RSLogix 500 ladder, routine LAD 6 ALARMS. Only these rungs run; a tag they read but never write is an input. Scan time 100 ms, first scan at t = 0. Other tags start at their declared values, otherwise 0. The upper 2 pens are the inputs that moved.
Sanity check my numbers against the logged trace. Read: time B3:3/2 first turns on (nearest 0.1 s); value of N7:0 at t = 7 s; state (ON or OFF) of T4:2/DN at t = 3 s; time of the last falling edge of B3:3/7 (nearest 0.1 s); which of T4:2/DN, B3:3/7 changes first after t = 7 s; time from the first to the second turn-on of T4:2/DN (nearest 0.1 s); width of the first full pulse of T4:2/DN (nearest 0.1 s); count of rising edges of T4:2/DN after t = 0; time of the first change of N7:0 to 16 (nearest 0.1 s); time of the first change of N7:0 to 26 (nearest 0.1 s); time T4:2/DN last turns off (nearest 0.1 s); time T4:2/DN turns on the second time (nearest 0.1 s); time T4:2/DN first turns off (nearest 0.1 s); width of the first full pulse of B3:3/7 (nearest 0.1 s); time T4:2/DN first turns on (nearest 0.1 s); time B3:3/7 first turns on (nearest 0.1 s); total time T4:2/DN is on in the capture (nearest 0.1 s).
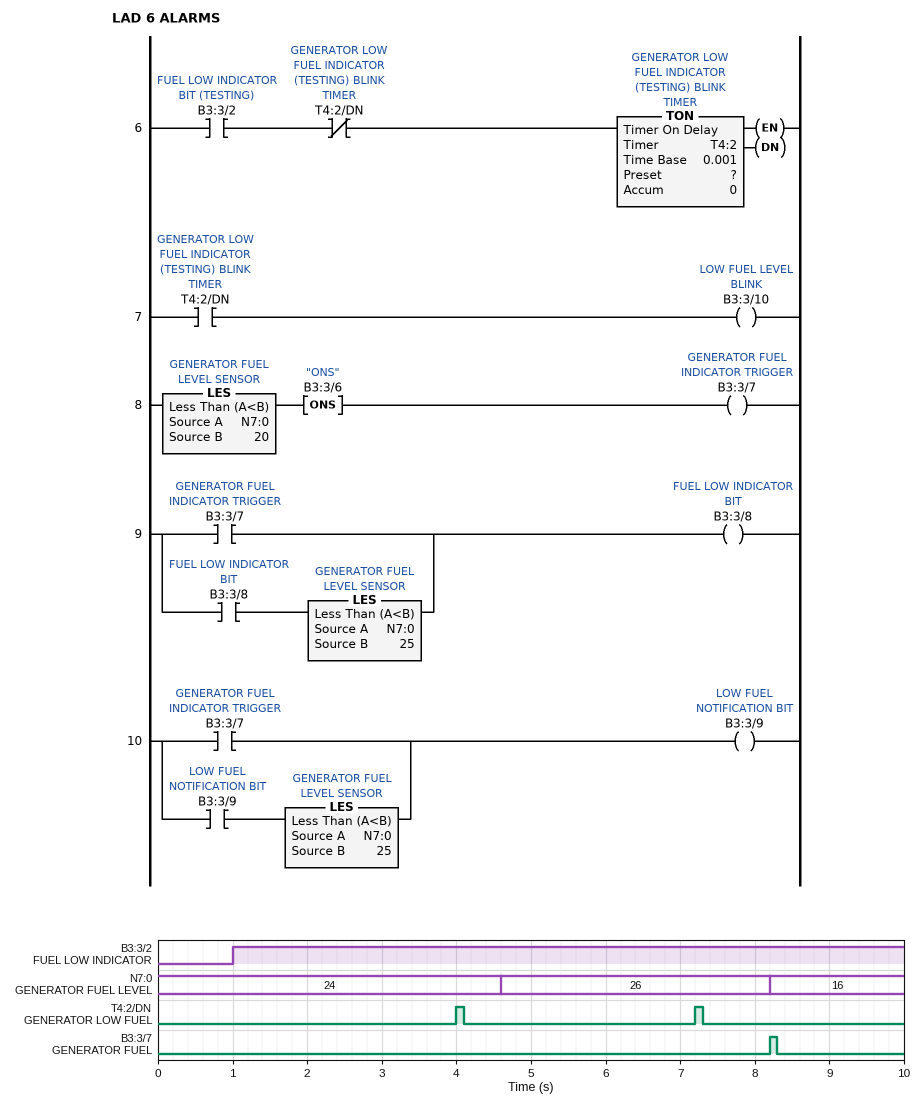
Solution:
1.0 s
26
OFF
8.3 s
T4:2/DN
3.2 s
0.1 s
2
8.2 s
4.6 s
7.3 s
7.2 s
4.1 s
0.1 s
4.0 s
8.2 s
0.2 s
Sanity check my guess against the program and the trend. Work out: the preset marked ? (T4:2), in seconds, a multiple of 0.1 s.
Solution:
3.0 s
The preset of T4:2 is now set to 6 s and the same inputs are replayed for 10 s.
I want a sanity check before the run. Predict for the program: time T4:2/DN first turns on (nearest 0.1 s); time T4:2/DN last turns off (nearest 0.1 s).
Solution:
7.0 s
7.1 s
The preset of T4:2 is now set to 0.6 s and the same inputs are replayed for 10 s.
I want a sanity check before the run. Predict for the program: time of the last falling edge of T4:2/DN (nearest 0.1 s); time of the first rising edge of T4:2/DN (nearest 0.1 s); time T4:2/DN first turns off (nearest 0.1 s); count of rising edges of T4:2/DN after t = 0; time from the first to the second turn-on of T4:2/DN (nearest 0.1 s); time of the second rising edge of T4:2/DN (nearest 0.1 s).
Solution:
9.7 s
1.6 s
1.7 s
11
0.8 s
2.4 s
